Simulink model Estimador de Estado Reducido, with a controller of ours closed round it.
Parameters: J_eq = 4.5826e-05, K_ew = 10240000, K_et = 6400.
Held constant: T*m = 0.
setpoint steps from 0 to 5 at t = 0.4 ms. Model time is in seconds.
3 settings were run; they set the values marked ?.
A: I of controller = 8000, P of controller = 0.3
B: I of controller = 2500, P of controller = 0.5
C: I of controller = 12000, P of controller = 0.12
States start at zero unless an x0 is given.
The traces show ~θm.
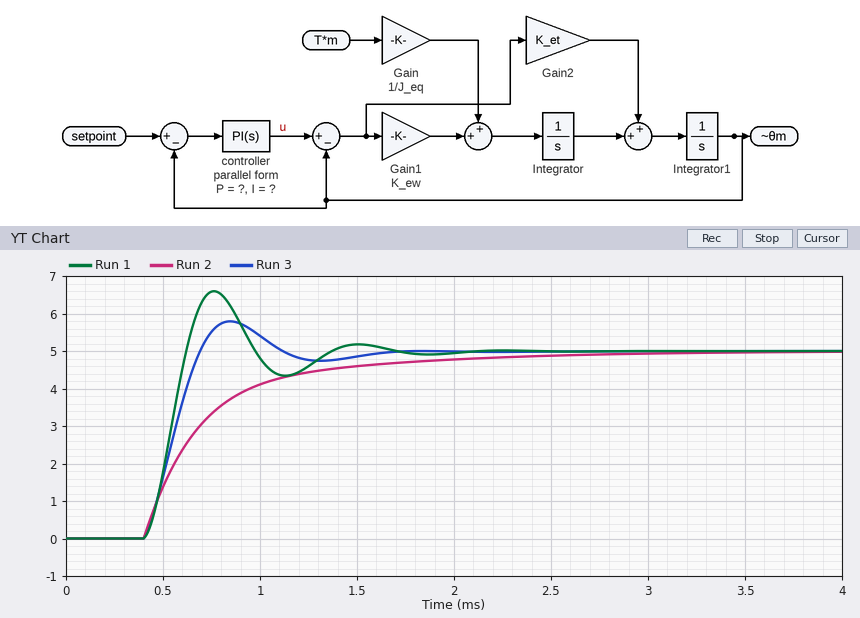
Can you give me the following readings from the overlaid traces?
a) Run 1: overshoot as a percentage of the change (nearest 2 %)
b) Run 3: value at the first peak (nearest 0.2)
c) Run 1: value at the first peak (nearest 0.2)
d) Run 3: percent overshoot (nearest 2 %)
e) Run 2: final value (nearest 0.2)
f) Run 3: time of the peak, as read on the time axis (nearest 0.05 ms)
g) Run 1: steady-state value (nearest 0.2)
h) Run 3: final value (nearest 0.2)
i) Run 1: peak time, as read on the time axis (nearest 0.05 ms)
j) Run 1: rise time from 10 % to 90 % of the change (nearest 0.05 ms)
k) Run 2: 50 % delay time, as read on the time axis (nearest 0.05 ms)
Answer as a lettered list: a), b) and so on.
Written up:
a) 32 %
b) 5.8
c) 6.6
d) 16 %
e) 5.0
f) 0.85 ms
g) 5.0
h) 5.0
i) 0.75 ms
j) 0.15 ms
k) 0.60 ms
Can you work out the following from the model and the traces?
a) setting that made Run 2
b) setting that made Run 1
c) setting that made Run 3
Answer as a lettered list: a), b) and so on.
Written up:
a) B
b) C
c) A
